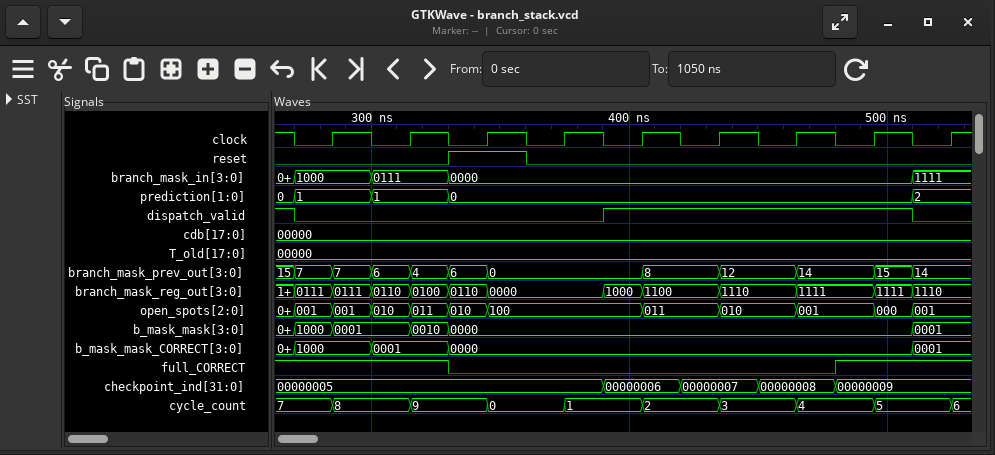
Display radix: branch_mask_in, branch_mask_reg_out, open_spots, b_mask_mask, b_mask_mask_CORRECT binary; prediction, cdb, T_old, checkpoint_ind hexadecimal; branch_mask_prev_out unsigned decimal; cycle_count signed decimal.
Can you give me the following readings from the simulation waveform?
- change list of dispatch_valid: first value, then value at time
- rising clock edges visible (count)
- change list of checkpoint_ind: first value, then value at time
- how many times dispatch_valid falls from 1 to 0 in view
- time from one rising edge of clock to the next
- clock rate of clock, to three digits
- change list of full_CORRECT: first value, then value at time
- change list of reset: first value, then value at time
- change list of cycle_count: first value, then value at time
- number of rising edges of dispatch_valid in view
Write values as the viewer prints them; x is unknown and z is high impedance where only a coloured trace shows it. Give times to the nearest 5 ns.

1, 0 at 270 ns, 1 at 390 ns, 0 at 510 ns
9
00000005, 00000006 at 390 ns, 00000007 at 420 ns, 00000008 at 450 ns, 00000009 at 480 ns
2
30 ns
33.3 MHz
1, 0 at 330 ns, 1 at 480 ns
0, 1 at 330 ns, 0 at 360 ns
7, 8 at 285 ns, 9 at 315 ns, 0 at 345 ns, 1 at 375 ns, 2 at 405 ns, 3 at 435 ns, 4 at 465 ns, 5 at 495 ns, 6 at 525 ns
1
